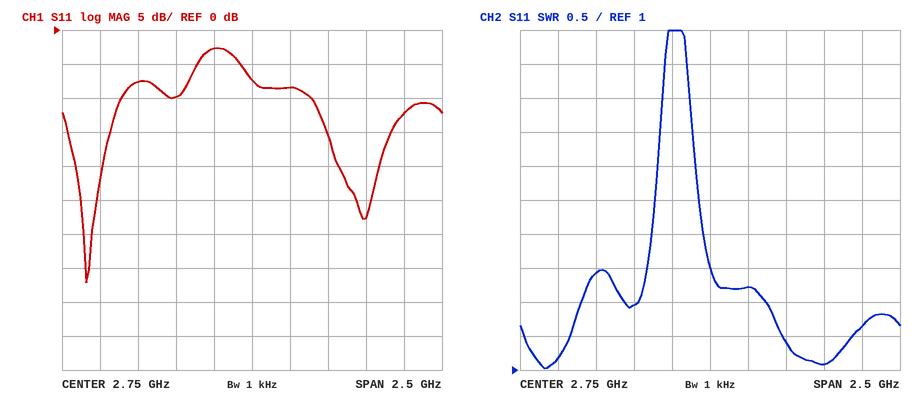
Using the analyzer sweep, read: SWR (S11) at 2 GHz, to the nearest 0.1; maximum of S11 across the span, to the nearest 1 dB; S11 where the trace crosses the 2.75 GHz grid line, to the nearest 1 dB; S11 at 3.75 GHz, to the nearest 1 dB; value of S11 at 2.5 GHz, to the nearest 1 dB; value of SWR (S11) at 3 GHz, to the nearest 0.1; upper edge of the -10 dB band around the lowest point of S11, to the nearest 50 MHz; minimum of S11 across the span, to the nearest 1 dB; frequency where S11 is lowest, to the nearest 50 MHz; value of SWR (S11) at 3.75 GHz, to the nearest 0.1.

2.4
-3 dB
-7 dB
-12 dB
-3 dB
2.2
1.90 GHz
-37 dB
1.65 GHz
1.6
